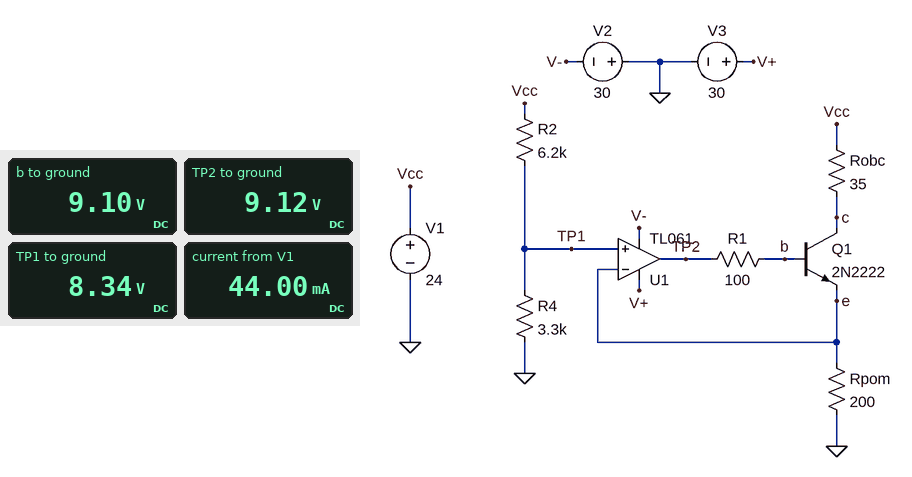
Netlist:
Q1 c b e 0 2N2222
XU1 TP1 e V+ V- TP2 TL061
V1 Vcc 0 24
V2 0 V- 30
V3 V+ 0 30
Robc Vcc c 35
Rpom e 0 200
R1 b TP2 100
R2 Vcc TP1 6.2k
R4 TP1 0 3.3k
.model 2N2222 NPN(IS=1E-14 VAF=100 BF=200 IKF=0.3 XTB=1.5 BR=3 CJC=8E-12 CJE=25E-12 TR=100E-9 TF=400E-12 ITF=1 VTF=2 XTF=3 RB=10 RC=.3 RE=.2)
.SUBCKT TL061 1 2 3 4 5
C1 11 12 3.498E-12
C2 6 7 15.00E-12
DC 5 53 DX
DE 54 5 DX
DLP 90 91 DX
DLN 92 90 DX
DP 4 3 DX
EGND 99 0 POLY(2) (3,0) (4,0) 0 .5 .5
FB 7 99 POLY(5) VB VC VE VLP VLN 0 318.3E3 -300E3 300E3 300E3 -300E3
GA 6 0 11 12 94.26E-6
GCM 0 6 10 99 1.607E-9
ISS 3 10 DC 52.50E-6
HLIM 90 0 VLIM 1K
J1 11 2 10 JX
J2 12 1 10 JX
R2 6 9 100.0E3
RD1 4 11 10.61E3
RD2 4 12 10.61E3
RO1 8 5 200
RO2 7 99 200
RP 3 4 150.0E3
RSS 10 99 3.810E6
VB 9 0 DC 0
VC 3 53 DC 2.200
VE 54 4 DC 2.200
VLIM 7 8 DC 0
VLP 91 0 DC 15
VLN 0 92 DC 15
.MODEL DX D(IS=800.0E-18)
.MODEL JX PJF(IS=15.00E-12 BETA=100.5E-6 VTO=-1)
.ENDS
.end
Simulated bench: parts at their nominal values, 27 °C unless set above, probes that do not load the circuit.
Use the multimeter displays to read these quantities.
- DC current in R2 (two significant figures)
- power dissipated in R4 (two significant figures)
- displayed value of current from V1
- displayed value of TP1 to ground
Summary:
2.5 mA
21 mW
44.00 mA
8.34 V
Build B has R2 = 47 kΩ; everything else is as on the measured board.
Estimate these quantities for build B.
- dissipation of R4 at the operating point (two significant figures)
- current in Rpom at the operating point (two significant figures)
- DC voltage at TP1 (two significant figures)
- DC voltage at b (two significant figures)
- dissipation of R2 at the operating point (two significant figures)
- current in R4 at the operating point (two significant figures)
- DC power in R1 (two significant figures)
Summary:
750 µW
7.9 mA
1.6 V
2.3 V
11 mW
480 µA
110 nW
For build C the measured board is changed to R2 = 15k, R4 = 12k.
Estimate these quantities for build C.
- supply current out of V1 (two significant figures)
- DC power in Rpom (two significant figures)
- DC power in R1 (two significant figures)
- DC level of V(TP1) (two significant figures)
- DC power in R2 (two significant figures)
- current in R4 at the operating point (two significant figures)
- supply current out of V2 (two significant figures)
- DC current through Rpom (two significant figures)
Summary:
54 mA
570 mW
7.7 µW
11 V
12 mW
890 µA
450 µA
53 mA
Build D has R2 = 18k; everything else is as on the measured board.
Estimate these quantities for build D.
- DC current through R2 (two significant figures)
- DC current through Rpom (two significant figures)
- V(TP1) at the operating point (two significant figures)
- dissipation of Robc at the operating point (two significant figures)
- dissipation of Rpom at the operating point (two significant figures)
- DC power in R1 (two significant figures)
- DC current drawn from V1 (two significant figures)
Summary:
1.1 mA
19 mA
3.7 V
12 mW
69 mW
670 nW
20 mA
